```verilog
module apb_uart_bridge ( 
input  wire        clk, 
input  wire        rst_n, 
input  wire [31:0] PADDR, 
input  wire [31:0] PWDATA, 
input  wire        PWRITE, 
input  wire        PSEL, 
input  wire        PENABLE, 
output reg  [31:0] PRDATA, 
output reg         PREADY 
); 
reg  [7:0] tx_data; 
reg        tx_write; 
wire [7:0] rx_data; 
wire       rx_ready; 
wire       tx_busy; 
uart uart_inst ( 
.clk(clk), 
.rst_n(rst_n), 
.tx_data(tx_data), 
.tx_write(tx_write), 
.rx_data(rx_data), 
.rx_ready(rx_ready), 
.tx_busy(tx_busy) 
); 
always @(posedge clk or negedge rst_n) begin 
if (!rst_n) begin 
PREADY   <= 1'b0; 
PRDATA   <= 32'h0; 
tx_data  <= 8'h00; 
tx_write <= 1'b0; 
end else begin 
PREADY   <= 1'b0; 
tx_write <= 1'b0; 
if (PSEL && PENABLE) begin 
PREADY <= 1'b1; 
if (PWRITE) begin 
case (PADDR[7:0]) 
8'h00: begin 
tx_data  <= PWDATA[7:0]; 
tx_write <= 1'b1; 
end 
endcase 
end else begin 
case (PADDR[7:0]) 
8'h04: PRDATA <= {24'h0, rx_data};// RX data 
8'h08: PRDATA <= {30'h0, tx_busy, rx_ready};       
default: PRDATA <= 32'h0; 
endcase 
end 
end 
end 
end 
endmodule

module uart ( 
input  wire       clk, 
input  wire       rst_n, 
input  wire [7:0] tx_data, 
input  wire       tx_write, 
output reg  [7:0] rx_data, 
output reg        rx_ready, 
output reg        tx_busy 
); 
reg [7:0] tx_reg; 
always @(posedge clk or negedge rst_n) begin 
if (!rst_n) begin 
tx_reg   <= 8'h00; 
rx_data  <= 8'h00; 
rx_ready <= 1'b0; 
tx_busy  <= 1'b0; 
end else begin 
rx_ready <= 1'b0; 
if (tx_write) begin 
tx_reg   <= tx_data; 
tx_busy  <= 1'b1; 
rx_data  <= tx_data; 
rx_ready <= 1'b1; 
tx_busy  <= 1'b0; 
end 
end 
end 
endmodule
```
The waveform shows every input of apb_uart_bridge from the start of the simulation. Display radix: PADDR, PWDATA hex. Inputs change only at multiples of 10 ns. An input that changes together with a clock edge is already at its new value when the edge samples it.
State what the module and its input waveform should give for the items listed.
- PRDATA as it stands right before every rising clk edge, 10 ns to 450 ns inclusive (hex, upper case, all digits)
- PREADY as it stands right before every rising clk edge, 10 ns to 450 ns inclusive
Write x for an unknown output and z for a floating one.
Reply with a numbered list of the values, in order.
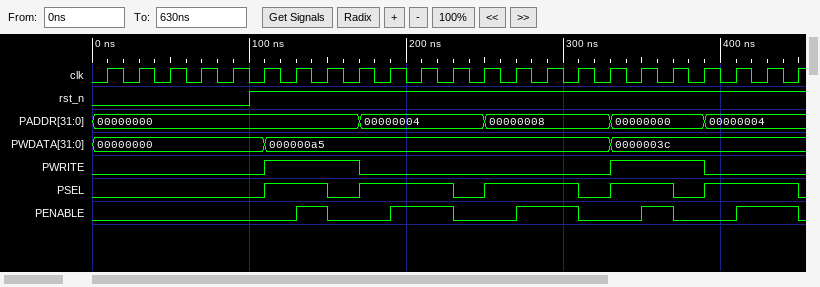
1. 00000000, 00000000, 00000000, 00000000, 00000000, 00000000, 00000000, 00000000, 00000000, 00000000, 000000A5, 000000A5, 000000A5, 000000A5, 00000000, 00000000, 00000000, 00000000, 00000000, 00000000, 00000000, 0000003C, 0000003C
2. 0 0 0 0 0 0 0 1 0 0 1 1 0 0 1 1 0 0 1 0 0 1 1
